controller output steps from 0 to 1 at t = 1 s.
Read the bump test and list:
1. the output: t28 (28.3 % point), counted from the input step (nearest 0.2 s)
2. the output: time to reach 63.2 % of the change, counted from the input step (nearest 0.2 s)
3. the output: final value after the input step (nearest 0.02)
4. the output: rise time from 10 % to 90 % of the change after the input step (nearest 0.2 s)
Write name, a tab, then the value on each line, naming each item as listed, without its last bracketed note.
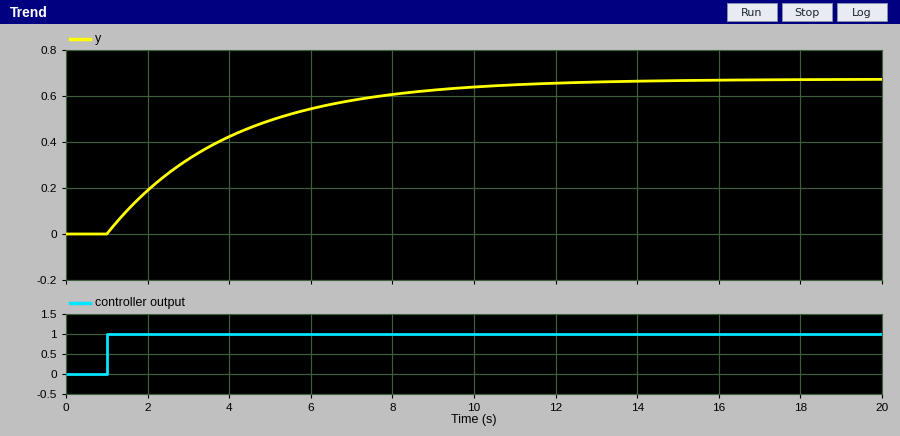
the output: t28 (28.3 % point), counted from the input step	1.0 s
the output: time to reach 63.2 % of the change, counted from the input step	3.0 s
the output: final value after the input step	0.68
the output: rise time from 10 % to 90 % of the change after the input step	6.6 s
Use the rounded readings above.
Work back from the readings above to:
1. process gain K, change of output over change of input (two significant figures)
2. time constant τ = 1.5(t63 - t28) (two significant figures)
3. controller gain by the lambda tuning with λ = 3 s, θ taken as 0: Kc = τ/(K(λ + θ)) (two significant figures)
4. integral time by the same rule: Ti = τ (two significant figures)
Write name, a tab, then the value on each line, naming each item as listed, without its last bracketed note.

process gain K, change of output over change of input	0.68
time constant τ = 1.5(t63 - t28)	3.0 s
controller gain by the lambda tuning with λ = 3 s, θ taken as 0: Kc = τ/(K(λ + θ))	1.5
integral time by the same rule: Ti = τ	3.0 s
